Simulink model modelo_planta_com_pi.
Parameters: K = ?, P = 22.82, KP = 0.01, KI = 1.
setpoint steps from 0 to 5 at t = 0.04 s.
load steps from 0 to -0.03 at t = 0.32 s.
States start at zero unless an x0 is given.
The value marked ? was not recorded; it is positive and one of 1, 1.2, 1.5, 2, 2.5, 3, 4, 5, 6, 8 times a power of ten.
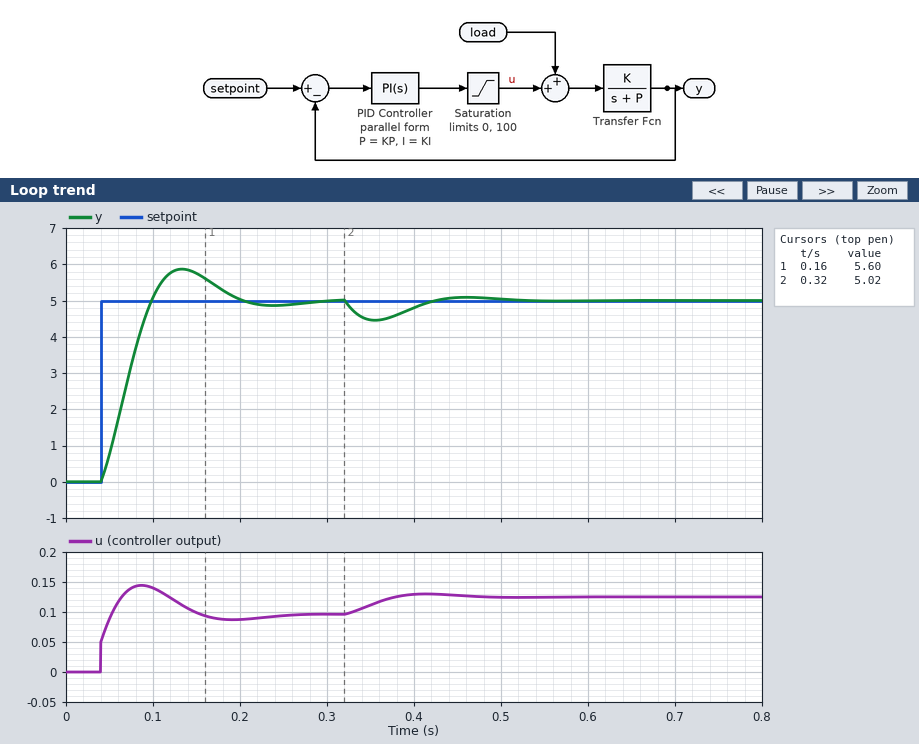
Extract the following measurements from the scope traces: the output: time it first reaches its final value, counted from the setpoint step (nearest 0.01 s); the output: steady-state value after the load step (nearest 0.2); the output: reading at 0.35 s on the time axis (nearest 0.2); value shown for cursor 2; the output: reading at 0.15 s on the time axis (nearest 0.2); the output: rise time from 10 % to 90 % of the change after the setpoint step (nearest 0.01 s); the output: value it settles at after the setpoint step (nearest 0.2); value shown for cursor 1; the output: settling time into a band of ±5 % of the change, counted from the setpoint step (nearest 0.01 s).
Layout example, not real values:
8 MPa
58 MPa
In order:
0.06 s
5.0
4.4
5.02
5.8
0.04 s
5.0
5.60
0.14 s
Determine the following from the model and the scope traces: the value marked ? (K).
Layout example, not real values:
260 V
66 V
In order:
1200
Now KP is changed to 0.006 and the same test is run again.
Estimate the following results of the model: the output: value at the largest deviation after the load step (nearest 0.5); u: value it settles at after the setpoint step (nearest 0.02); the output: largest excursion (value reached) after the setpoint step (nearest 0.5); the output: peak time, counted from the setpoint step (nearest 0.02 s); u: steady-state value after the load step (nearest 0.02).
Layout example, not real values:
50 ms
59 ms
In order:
4.5
0.10
6.0
0.10 s
0.12
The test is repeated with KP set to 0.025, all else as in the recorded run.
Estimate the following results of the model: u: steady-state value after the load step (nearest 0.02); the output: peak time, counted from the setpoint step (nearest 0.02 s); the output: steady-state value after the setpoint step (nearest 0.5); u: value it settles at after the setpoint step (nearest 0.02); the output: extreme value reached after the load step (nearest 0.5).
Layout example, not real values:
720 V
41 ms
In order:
0.12
0.10 s
5.0
0.10
4.5
